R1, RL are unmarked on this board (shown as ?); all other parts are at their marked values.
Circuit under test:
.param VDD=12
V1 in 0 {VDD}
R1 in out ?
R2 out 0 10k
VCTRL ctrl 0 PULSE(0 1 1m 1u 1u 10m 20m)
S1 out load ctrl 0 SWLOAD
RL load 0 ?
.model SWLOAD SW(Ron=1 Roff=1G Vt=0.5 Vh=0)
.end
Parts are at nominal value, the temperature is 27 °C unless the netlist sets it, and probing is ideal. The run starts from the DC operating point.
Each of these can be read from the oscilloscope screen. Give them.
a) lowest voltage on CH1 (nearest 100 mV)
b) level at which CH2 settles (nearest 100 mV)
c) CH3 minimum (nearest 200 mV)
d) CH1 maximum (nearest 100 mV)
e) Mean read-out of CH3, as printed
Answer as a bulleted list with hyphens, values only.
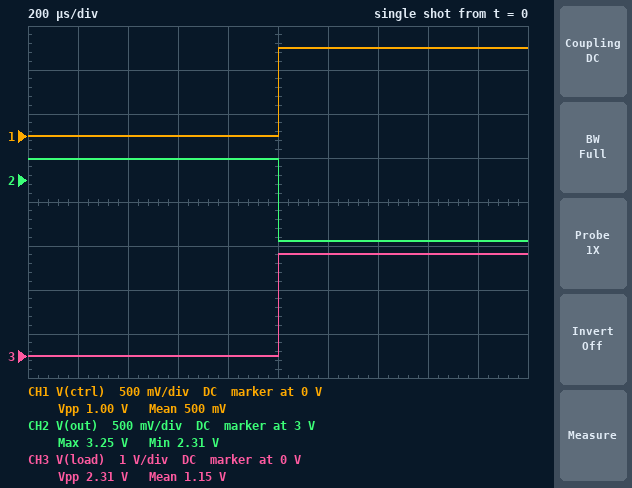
- 0 V
- 2.3 V
- 0 V
- 1.0 V
- 1.15 V
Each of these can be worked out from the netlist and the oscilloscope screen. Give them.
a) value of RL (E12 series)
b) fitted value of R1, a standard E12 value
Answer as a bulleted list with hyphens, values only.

- 18 kΩ
- 27 kΩ
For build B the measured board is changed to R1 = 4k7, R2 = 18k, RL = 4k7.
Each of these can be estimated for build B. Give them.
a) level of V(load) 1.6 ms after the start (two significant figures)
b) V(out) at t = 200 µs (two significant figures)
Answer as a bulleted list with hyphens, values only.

- 5.3 V
- 9.5 V
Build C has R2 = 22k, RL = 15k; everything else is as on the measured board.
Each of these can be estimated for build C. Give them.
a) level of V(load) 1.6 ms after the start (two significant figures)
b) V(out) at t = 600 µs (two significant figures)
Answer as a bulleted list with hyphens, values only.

- 3.0 V
- 5.4 V
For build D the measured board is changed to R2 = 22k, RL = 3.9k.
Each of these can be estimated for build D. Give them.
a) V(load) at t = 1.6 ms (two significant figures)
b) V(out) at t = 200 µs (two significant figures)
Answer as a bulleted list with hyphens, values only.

- 1.3 V
- 5.4 V
